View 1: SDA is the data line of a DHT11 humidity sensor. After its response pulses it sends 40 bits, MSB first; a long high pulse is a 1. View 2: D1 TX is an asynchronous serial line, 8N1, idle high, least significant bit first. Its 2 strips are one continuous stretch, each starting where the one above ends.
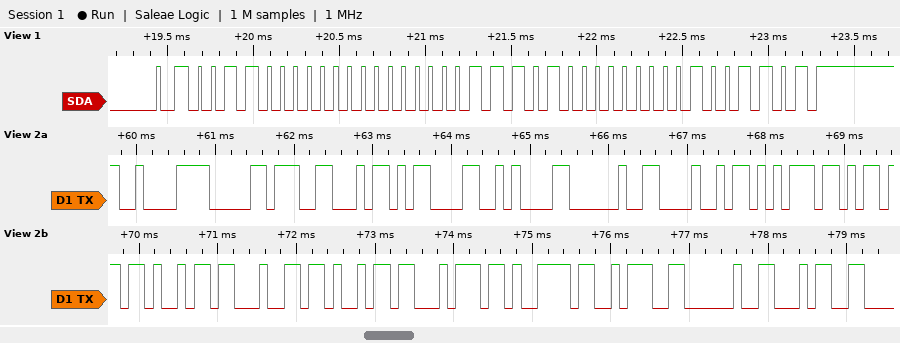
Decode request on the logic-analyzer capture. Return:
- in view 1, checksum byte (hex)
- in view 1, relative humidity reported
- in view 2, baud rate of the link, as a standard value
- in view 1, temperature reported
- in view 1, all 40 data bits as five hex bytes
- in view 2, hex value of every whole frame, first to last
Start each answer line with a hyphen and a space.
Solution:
- 0x4D
- 48 %
- 9600 baud
- 29.0 °C
- 30 00 1D 00 4D
- 0xC2 0xB0 0x46 0x0D 0x0A 0x20 0x48 0x75 0x6D 0x69 0x64 0x69 0x74 0x79 0x3A 0x20 0x34
